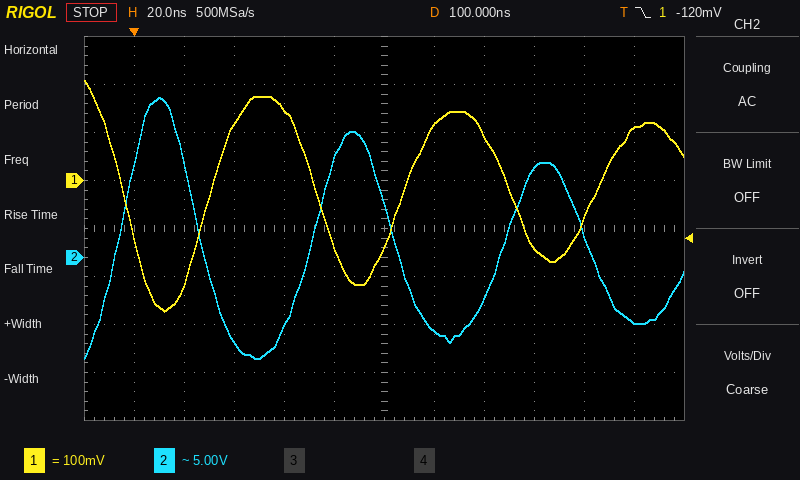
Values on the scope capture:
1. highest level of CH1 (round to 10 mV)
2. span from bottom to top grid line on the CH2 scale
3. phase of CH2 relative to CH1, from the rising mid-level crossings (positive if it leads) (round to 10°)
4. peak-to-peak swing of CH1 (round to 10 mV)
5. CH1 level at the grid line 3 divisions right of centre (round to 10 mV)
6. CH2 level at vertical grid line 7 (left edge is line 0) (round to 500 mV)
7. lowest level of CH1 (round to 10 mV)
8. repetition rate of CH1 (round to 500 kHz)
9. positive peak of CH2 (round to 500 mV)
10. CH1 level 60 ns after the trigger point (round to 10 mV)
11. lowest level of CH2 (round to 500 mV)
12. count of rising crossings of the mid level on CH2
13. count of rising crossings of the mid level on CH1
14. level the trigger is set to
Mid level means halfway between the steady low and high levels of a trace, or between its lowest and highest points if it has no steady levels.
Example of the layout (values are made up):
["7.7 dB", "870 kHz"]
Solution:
["210 mV", "40 V", "+160°", "480 mV", "-140 mV", "-7.5 V", "-270 mV", "13.0 MHz", "16.5 V", "150 mV", "-10.5 V", "3", "3", "-120 mV"]
